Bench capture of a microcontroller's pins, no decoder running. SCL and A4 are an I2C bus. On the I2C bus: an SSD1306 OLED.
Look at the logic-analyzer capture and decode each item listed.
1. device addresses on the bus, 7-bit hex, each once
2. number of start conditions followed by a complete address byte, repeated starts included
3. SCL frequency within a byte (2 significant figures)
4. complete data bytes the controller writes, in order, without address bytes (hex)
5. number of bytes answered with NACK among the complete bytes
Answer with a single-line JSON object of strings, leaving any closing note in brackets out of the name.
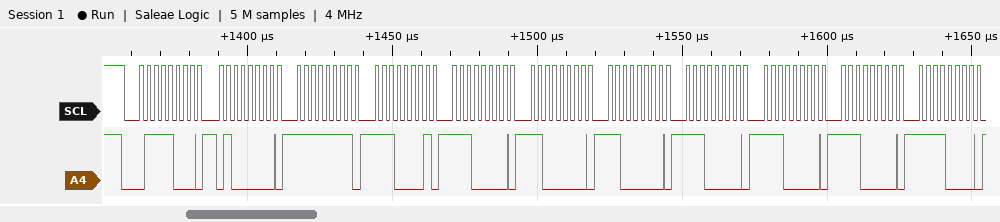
{"device addresses on the bus, 7-bit hex, each once": "0x3C", "number of start conditions followed by a complete address byte, repeated starts included": "1", "SCL frequency within a byte": "400 kHz", "complete data bytes the controller writes, in order, without address bytes": "40 FF E1 E0 C0 C0 E0 E0 E0 F0", "number of bytes answered with NACK among the complete bytes": "0"}
